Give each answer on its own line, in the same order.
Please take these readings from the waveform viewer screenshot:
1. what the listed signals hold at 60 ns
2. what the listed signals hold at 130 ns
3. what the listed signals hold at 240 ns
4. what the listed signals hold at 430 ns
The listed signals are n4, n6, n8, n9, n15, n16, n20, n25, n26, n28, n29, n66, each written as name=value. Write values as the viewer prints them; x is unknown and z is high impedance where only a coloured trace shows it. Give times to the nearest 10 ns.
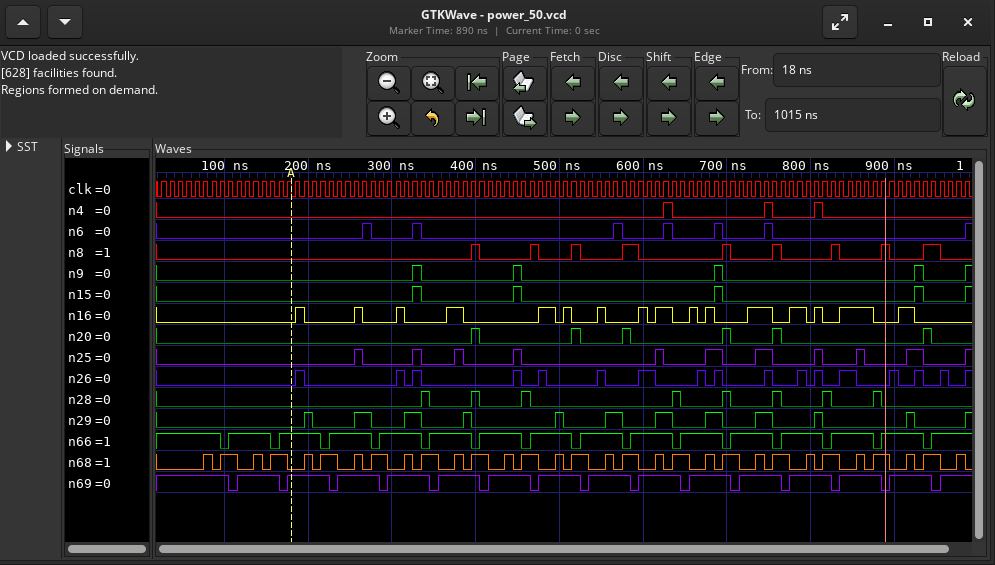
n4=0, n6=0, n8=0, n9=0, n15=0, n16=0, n20=0, n25=0, n26=0, n28=0, n29=0, n66=1
n4=0, n6=0, n8=0, n9=0, n15=0, n16=0, n20=0, n25=0, n26=0, n28=0, n29=0, n66=1
n4=0, n6=0, n8=0, n9=0, n15=0, n16=0, n20=0, n25=0, n26=0, n28=0, n29=0, n66=1
n4=0, n6=0, n8=0, n9=0, n15=0, n16=0, n20=0, n25=0, n26=0, n28=0, n29=0, n66=1
